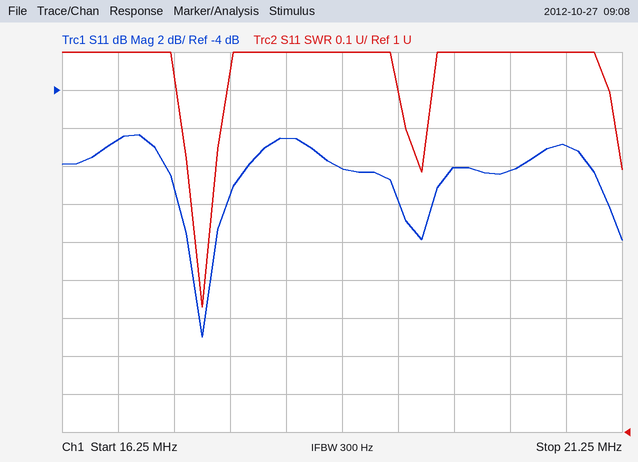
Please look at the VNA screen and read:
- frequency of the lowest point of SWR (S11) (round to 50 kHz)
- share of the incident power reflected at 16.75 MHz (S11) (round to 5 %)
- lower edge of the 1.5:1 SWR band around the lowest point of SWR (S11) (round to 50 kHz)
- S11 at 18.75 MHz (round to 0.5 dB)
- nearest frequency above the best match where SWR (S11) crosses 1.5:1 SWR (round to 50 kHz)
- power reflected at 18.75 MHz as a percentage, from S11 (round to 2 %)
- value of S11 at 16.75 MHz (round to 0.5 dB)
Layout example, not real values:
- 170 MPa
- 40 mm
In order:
- 17.50 MHz
- 20 %
- 17.45 MHz
- -8.0 dB
- 17.55 MHz
- 16 %
- -6.5 dB
